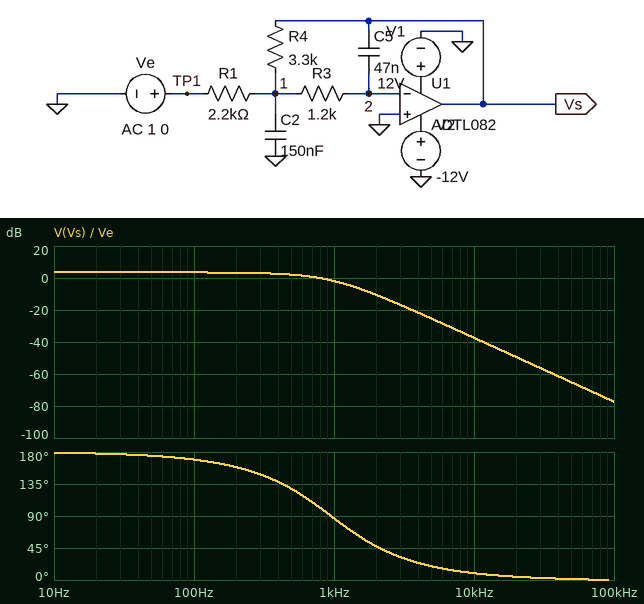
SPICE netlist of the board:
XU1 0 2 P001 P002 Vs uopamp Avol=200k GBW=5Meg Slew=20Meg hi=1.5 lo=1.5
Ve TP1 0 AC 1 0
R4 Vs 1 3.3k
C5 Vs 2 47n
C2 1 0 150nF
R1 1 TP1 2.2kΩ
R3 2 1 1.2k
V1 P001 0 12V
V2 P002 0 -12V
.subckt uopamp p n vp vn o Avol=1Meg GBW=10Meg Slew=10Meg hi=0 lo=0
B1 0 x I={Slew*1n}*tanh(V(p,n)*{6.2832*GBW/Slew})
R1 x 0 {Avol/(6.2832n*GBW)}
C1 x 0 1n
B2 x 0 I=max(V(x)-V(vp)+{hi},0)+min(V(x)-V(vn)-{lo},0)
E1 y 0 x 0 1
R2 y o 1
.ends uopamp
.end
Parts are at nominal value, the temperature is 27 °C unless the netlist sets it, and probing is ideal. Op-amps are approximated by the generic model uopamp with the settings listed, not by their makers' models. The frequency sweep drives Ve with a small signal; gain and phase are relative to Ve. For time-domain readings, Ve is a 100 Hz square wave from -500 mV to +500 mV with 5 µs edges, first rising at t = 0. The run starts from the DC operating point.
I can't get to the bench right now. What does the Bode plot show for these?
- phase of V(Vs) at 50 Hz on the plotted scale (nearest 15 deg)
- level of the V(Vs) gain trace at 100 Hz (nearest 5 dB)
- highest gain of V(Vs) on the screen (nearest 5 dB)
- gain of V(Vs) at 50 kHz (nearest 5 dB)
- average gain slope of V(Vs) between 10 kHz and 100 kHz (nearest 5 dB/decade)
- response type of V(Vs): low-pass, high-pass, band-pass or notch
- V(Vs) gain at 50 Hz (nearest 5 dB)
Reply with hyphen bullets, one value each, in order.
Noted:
- 180 deg
- 5 dB
- 5 dB
- -65 dB
- -40 dB/decade
- low-pass
- 5 dB
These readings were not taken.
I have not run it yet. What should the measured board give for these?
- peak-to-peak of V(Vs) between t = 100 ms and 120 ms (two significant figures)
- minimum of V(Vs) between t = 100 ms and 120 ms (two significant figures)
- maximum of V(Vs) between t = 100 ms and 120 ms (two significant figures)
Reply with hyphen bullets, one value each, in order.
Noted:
- 1.5 V
- -750 mV
- 750 mV
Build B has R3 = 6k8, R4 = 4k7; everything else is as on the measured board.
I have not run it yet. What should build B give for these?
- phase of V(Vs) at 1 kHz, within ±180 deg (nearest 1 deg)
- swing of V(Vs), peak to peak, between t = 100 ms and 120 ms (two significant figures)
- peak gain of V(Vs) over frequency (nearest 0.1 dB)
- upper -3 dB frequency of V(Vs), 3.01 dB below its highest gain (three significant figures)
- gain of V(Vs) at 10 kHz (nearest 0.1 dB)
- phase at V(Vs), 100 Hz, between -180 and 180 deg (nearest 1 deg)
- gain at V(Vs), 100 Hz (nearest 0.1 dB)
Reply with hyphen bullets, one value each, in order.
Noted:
- 44 deg
- 2.1 V
- 6.6 dB
- 152 Hz
- -52.4 dB
- 140 deg
- 5.1 dB
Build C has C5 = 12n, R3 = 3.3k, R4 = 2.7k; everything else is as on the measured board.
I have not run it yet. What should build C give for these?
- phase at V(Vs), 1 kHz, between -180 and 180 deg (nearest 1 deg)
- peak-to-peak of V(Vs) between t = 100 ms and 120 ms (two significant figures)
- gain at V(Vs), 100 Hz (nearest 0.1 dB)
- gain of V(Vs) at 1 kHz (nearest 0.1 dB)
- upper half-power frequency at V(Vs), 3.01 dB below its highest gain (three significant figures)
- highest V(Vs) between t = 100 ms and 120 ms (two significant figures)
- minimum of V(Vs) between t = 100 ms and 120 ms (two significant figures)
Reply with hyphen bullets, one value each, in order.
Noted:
- 116 deg
- 1.7 V
- 1.8 dB
- 3.3 dB
- 1.48 kHz
- 840 mV
- -840 mV
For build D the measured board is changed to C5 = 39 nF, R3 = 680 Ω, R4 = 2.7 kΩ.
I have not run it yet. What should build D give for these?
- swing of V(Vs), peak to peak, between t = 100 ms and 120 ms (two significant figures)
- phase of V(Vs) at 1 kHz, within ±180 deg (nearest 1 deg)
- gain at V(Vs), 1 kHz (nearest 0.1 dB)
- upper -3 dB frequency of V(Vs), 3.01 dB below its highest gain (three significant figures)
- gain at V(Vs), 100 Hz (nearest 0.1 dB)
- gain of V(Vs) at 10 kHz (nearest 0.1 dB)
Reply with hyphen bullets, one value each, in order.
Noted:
- 1.3 V
- 119 deg
- 0.3 dB
- 1.35 kHz
- 1.8 dB
- -30.8 dB
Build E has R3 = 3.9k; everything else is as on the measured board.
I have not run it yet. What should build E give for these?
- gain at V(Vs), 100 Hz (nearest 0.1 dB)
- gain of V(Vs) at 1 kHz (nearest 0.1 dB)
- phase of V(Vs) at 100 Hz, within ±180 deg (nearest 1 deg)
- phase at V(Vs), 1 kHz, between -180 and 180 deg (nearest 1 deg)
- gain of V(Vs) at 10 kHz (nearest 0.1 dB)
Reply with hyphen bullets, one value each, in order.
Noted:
- 3.2 dB
- -9.8 dB
- 158 deg
- 56 deg
- -47.6 dB
